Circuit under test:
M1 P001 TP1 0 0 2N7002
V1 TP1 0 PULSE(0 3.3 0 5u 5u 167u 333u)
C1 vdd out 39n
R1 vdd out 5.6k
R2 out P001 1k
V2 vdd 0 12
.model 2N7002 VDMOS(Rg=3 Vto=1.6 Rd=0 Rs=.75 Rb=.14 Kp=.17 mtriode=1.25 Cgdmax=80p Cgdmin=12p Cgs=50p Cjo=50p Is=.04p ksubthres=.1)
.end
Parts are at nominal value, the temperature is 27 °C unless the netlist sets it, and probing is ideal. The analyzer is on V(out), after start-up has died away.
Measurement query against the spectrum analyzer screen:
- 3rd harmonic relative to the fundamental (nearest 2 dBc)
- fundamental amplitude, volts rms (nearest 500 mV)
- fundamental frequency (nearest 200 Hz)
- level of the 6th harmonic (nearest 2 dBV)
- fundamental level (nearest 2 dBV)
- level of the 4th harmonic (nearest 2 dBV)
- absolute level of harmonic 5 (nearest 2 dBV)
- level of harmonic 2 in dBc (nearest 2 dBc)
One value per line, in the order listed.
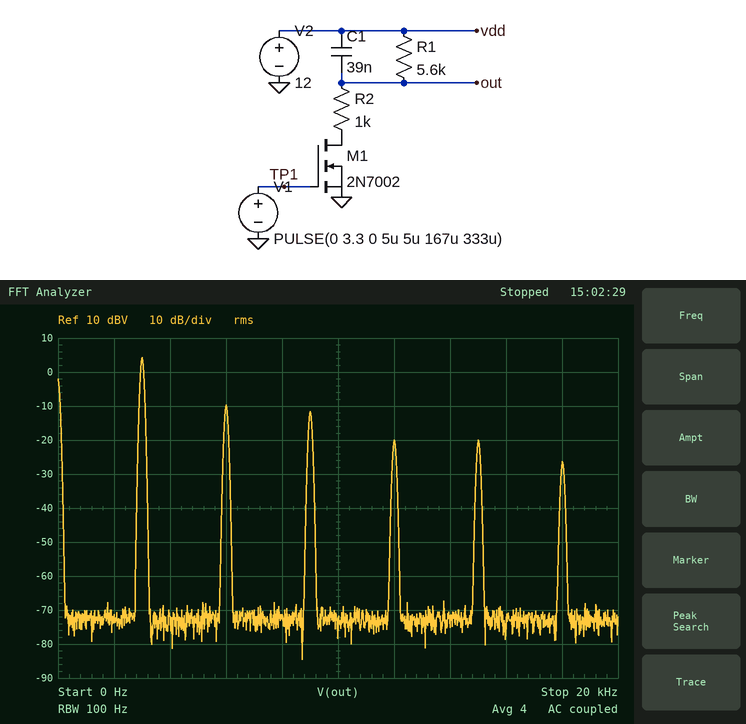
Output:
-16 dBc
1.5 V
3.0 kHz
-26 dBV
4 dBV
-20 dBV
-20 dBV
-14 dBc
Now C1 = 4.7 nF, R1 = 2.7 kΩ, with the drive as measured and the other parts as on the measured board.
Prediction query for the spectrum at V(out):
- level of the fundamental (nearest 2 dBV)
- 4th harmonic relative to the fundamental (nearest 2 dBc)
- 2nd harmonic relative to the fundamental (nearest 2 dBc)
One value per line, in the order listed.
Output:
12 dBV
-20 dBc
-18 dBc
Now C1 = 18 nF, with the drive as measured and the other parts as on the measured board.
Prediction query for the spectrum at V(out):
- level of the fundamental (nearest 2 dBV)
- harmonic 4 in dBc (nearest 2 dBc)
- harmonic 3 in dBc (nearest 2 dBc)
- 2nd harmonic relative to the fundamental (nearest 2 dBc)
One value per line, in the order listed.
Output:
8 dBV
-20 dBc
-14 dBc
-12 dBc
